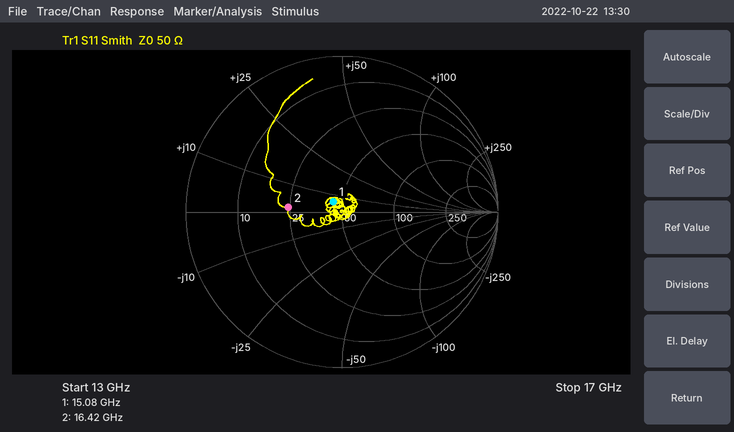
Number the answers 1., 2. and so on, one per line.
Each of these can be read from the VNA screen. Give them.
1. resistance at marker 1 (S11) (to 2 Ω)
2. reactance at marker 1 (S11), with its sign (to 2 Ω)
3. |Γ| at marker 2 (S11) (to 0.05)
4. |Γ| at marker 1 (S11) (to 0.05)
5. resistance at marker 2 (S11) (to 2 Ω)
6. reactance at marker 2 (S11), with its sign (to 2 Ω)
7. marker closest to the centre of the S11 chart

1. 44 Ω
2. +6 Ω
3. 0.35
4. 0.10
5. 24 Ω
6. +2 Ω
7. marker 1
